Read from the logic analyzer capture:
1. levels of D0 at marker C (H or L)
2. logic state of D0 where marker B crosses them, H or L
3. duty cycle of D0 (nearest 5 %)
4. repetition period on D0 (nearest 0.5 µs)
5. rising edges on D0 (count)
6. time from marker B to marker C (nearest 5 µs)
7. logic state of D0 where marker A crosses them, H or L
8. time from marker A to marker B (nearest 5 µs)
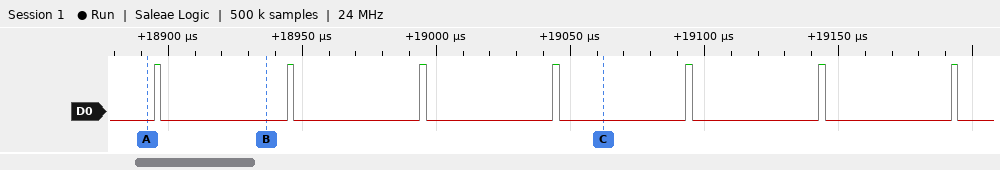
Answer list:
D0=L
D0=L
5 %
49.5 µs
7
125 µs
D0=L
45 µs
